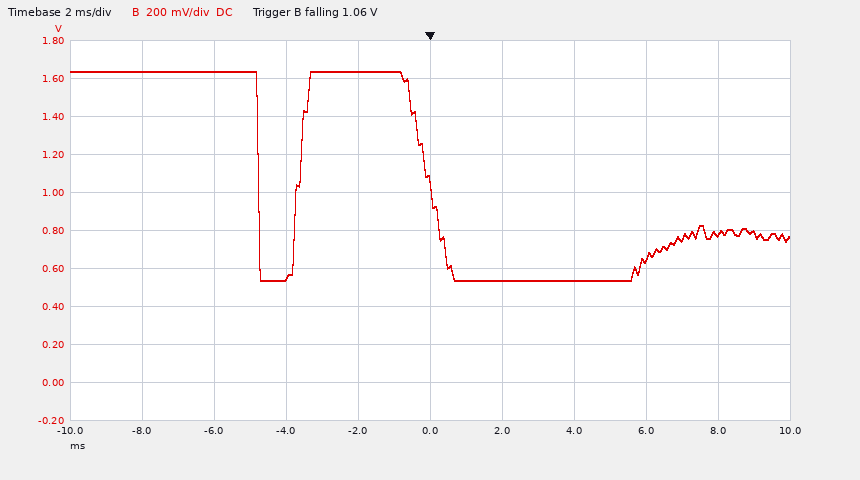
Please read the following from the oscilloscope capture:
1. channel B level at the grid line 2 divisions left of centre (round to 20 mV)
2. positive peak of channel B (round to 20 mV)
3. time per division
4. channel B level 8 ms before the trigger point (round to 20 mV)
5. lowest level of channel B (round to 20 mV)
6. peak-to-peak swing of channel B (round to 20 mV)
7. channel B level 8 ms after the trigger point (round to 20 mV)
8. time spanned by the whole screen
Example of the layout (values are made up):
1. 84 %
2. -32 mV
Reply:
1. 560 mV
2. 1.64 V
3. 2 ms
4. 1.64 V
5. 540 mV
6. 1.10 V
7. 780 mV
8. 20 ms
